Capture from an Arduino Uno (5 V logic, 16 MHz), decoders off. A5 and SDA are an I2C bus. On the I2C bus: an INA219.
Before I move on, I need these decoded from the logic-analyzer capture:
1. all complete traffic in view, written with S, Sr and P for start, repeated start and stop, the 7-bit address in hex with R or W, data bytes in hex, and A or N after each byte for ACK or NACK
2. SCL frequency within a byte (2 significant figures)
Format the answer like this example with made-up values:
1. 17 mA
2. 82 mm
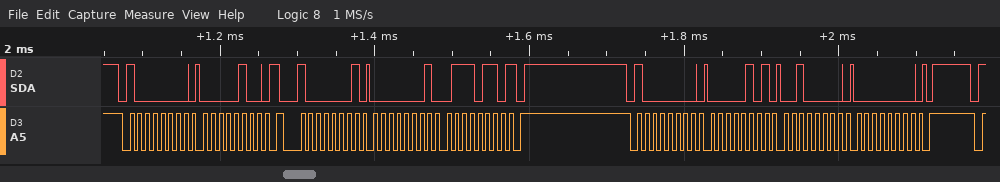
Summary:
1. S 40W A 04 A Sr 40R A 01 A 76 N P S 40W A 05 A 20 A 00 A P
2. 100 kHz
